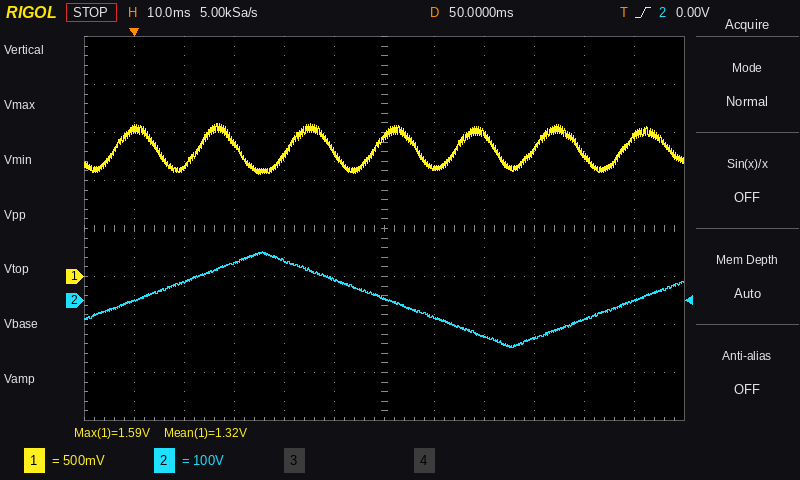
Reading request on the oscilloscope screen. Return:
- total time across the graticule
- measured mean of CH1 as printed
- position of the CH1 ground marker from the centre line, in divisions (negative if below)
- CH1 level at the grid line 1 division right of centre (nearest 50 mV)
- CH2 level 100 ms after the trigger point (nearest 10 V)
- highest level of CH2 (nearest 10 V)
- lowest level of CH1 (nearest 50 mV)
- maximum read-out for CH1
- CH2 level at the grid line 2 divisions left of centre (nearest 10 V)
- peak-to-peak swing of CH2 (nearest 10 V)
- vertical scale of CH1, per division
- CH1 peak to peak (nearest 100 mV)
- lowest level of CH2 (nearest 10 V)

120 ms
1.32 V
-1.0 div
1.15 V
0 V
100 V
1.05 V
1.59 V
80 V
200 V
500 mV
500 mV
-100 V
